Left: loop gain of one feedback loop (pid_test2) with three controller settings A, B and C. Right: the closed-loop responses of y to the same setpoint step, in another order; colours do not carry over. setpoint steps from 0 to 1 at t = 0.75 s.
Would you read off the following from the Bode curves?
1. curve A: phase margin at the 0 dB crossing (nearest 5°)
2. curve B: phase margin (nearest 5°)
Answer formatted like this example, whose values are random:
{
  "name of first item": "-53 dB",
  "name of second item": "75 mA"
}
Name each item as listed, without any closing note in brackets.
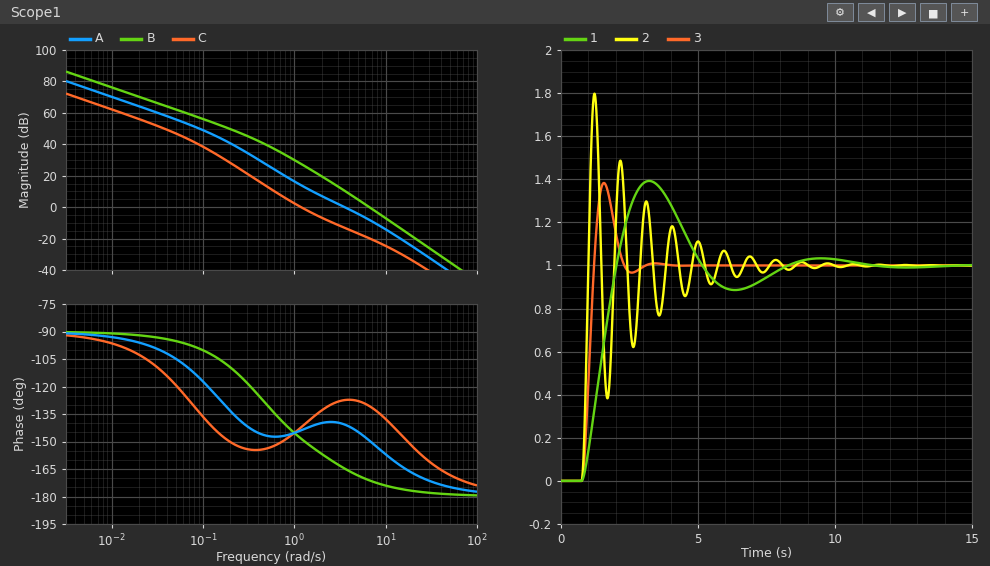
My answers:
{
  "curve A: phase margin at the 0 dB crossing": "40°",
  "curve B: phase margin": "10°"
}
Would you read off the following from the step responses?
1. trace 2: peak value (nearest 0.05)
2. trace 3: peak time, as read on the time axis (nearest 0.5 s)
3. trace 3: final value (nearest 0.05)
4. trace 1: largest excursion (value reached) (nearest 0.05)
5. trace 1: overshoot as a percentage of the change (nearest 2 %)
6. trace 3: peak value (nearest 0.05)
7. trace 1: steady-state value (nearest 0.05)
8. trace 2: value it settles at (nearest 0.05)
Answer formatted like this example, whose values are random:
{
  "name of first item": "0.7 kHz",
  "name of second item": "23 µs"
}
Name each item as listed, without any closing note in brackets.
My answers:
{
  "trace 2: peak value": "1.80",
  "trace 3: peak time, as read on the time axis": "1.5 s",
  "trace 3: final value": "1.00",
  "trace 1: largest excursion (value reached)": "1.40",
  "trace 1: overshoot as a percentage of the change": "40 %",
  "trace 3: peak value": "1.40",
  "trace 1: steady-state value": "1.00",
  "trace 2: value it settles at": "1.00"
}
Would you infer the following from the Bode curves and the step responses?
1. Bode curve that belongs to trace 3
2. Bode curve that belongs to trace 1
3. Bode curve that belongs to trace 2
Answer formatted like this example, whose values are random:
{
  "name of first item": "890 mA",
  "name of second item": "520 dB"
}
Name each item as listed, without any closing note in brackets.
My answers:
{
  "Bode curve that belongs to trace 3": "A",
  "Bode curve that belongs to trace 1": "C",
  "Bode curve that belongs to trace 2": "B"
}
